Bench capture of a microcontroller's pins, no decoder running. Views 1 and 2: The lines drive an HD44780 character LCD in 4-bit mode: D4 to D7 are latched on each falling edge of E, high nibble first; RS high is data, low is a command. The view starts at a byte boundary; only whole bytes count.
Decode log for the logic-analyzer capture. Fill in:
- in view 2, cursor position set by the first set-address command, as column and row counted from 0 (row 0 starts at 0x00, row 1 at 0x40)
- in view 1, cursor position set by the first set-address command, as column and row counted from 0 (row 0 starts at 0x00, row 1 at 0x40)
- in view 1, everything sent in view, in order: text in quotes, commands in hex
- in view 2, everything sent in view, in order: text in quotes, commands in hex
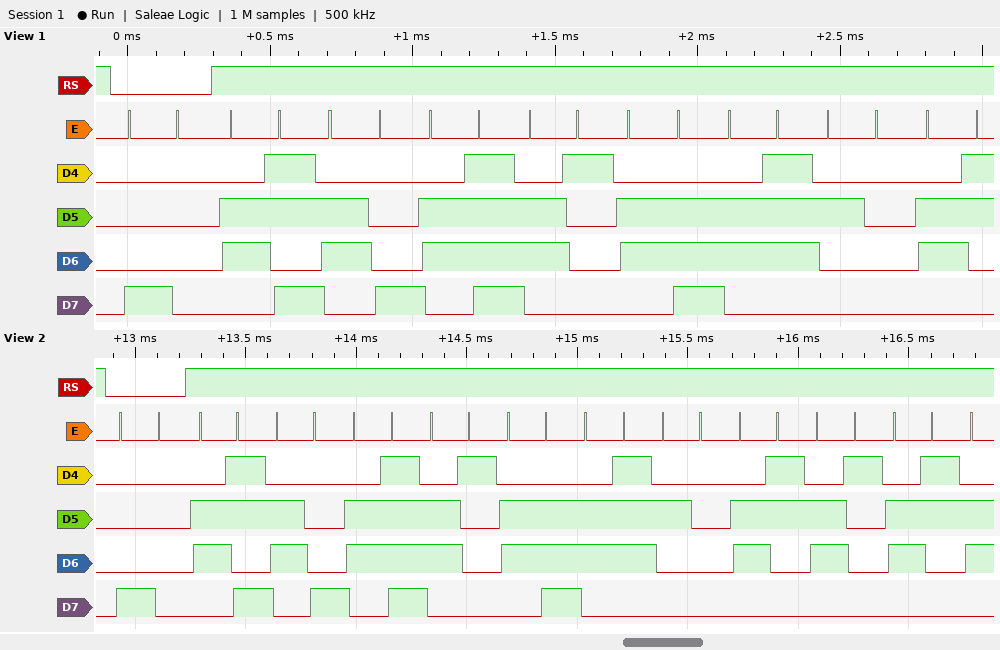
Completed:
column 0, row 0
column 0, row 0
0x80 "khoang c"
0x80 "khoang cac"
